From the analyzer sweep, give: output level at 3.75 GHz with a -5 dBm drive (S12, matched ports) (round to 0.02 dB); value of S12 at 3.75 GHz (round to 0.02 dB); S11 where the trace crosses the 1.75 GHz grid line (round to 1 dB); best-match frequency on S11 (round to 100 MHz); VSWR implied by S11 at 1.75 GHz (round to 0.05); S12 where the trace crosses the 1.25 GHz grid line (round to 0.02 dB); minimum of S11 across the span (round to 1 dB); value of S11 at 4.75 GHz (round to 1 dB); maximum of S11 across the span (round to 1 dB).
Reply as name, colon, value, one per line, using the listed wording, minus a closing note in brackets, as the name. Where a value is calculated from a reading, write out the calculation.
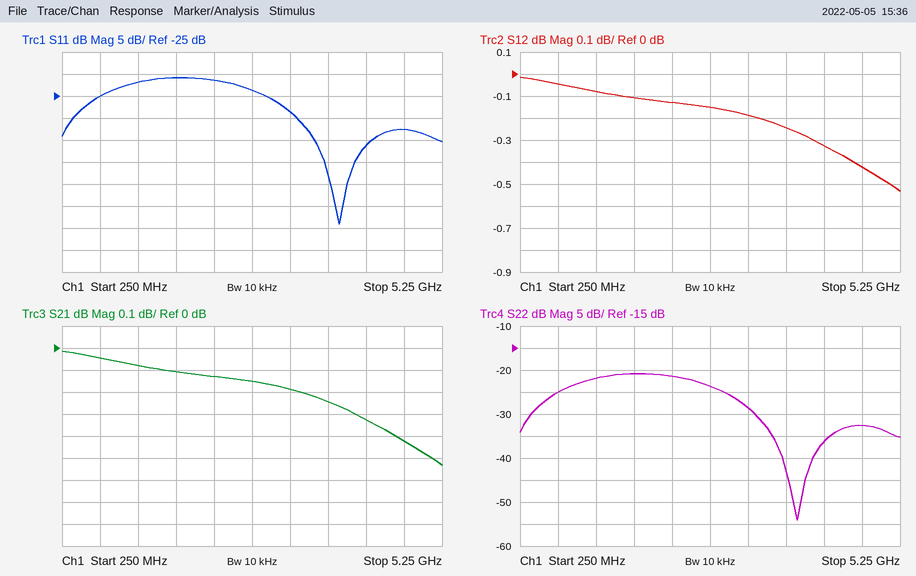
output level at 3.75 GHz with a -5 dBm drive (S12, matched ports): -5 dBm + (-0.24 dB) = -5.24 dBm
value of S12 at 3.75 GHz: -0.24 dB
S11 where the trace crosses the 1.75 GHz grid line: -21 dB
best-match frequency on S11: 3.9 GHz
VSWR implied by S11 at 1.75 GHz: |Γ| = 10^(-21/20) = 0.0891; VSWR = (1 + 0.0891)/(1 − 0.0891) ≈ 1.20
S12 where the trace crosses the 1.25 GHz grid line: -0.08 dB
minimum of S11 across the span: -54 dB
value of S11 at 4.75 GHz: -33 dB
maximum of S11 across the span: -21 dB
